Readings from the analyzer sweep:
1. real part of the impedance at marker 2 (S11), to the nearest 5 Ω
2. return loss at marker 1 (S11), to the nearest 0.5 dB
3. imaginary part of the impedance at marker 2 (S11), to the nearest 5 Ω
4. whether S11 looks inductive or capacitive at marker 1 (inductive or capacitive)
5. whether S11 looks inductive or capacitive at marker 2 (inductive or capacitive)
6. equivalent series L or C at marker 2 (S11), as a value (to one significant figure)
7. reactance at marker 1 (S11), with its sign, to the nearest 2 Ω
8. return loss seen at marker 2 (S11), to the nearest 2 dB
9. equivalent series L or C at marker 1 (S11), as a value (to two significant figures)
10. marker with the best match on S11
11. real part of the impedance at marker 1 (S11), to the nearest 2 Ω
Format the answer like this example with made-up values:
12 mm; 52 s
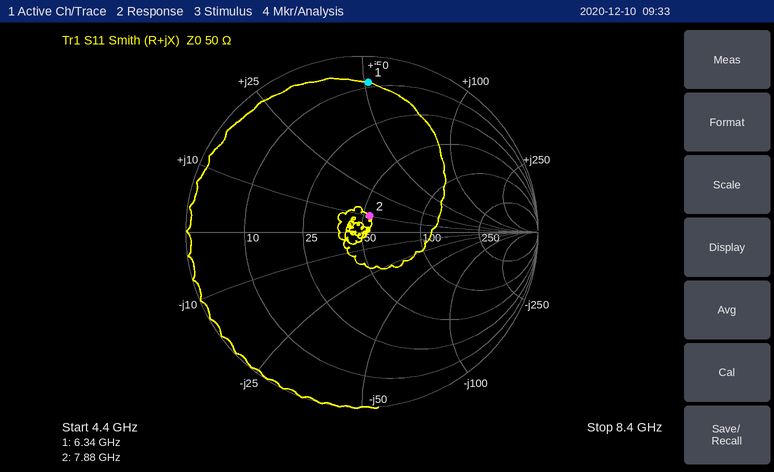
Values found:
55 Ω; 1.5 dB; +10 Ω; inductive; inductive; 200 pH; +52 Ω; 20 dB; 1.3 nH; marker 2; 8 Ω
